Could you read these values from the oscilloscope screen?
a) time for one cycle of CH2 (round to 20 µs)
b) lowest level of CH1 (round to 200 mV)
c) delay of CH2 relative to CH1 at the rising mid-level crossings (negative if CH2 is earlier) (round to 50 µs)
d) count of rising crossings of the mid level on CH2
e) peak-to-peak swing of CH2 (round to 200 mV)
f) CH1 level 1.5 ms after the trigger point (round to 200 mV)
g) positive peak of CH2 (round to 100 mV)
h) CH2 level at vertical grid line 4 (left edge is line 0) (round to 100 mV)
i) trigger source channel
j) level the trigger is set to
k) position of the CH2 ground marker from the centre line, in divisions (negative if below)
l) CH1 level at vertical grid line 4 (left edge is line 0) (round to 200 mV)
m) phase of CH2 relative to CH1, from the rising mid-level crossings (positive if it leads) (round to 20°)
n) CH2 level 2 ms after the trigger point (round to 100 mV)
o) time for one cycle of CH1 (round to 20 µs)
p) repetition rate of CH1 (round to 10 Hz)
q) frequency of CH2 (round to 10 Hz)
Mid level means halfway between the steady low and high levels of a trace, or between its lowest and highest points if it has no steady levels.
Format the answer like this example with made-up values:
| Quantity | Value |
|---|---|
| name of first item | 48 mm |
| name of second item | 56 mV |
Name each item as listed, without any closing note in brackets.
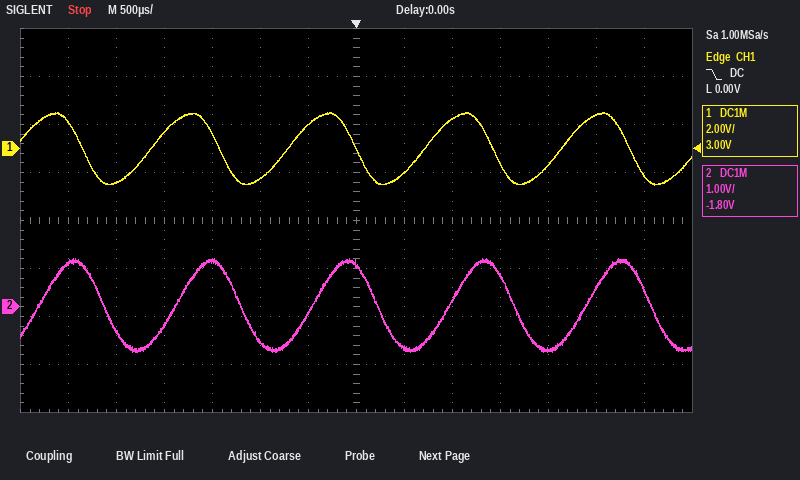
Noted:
| Quantity | Value |
|---|---|
| time for one cycle of CH2 | 1.42 ms |
| lowest level of CH1 | -1.6 V |
| delay of CH2 relative to CH1 at the rising mid-level crossings (negative if CH2 is earlier) | +250 µs |
| count of rising crossings of the mid level on CH2 | 5 |
| peak-to-peak swing of CH2 | 2.0 V |
| CH1 level 1.5 ms after the trigger point | -600 mV |
| positive peak of CH2 | 1.0 V |
| CH2 level at vertical grid line 4 (left edge is line 0) | 900 mV |
| trigger source channel | CH1 |
| level the trigger is set to | 0.00 V |
| position of the CH2 ground marker from the centre line, in divisions | -1.8 div |
| CH1 level at vertical grid line 4 (left edge is line 0) | 600 mV |
| phase of CH2 relative to CH1, from the rising mid-level crossings (positive if it leads) | -60° |
| CH2 level 2 ms after the trigger point | -900 mV |
| time for one cycle of CH1 | 1.42 ms |
| repetition rate of CH1 | 700 Hz |
| frequency of CH2 | 700 Hz |
